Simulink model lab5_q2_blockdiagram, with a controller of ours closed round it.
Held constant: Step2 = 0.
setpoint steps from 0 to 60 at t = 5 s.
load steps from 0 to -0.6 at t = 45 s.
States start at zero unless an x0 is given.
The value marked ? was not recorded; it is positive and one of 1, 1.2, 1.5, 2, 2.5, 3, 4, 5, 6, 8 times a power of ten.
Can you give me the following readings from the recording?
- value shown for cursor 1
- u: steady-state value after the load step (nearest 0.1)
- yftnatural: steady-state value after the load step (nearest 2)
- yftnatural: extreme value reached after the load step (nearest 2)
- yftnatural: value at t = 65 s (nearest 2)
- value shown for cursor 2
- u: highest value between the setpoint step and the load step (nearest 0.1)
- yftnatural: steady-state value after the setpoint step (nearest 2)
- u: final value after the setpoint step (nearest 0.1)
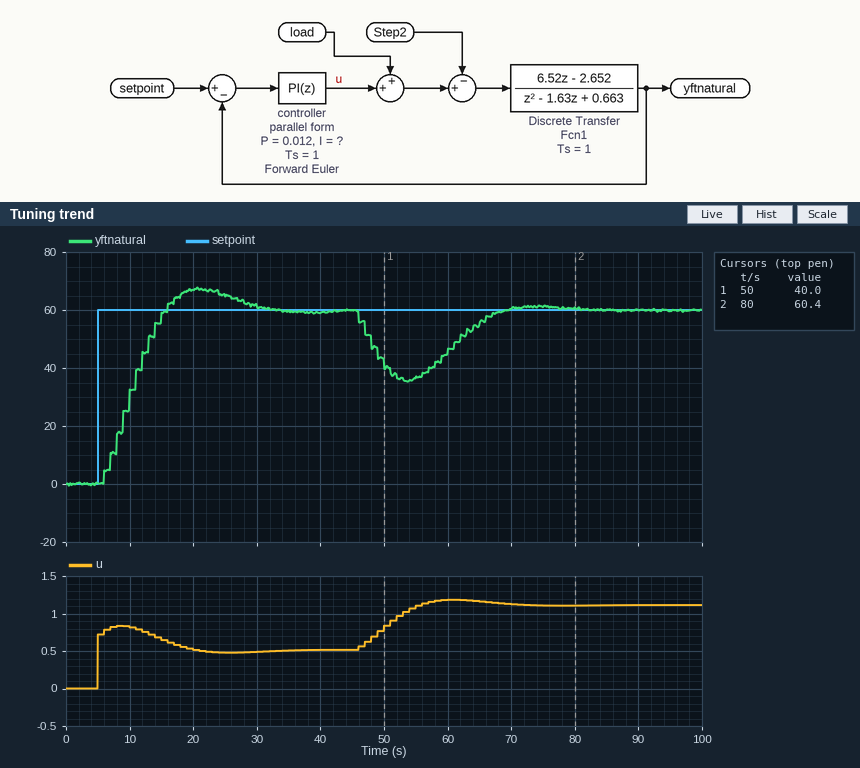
40.0
1.1
60
36
56
60.4
0.8
60
0.5
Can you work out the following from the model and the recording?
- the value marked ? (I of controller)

0.002
